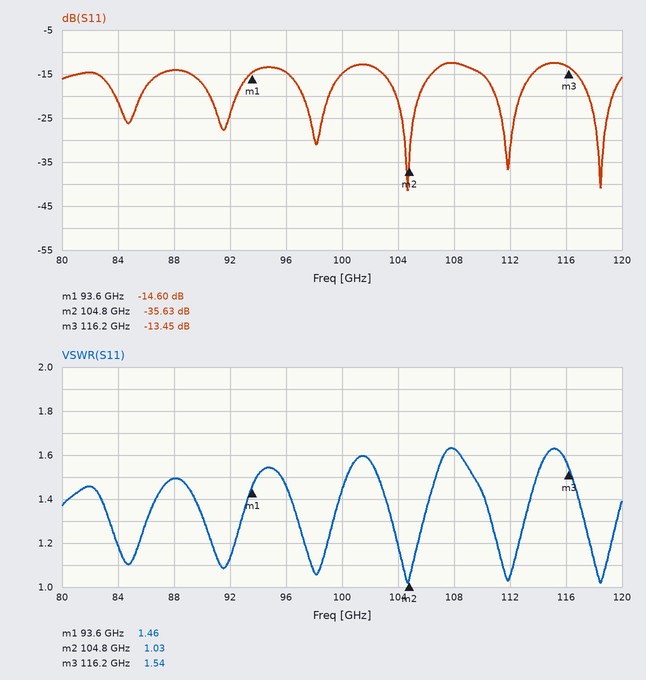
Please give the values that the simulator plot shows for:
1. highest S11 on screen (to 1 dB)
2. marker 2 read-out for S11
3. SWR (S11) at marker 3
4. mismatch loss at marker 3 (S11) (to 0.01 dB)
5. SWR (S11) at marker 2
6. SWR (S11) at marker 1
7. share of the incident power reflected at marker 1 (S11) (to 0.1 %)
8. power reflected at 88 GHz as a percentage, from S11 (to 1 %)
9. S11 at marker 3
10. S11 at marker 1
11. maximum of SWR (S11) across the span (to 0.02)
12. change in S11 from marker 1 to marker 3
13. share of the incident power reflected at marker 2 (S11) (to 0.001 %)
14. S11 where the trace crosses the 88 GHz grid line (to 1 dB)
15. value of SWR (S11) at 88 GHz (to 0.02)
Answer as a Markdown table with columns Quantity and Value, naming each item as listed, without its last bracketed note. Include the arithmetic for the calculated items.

| Quantity | Value |
|---|---|
| highest S11 on screen | -12 dB |
| marker 2 read-out for S11 | -35.63 dB |
| SWR (S11) at marker 3 | 1.54 |
| mismatch loss at marker 3 (S11) | −10 log10(1 − 10^(-13.45/10)) ≈ 0.20 dB |
| SWR (S11) at marker 2 | 1.03 |
| SWR (S11) at marker 1 | 1.46 |
| share of the incident power reflected at marker 1 (S11) | 10^(-14.6/10) ≈ 3.5 % |
| power reflected at 88 GHz as a percentage, from S11 | 10^(-14/10) ≈ 4 % |
| S11 at marker 3 | -13.45 dB |
| S11 at marker 1 | -14.60 dB |
| maximum of SWR (S11) across the span | 1.64 |
| change in S11 from marker 1 to marker 3 | -13.45 − (-14.6) = 1.15 dB |
| share of the incident power reflected at marker 2 (S11) | 10^(-35.63/10) ≈ 0.027 % |
| S11 where the trace crosses the 88 GHz grid line | -14 dB |
| value of SWR (S11) at 88 GHz | 1.50 |
